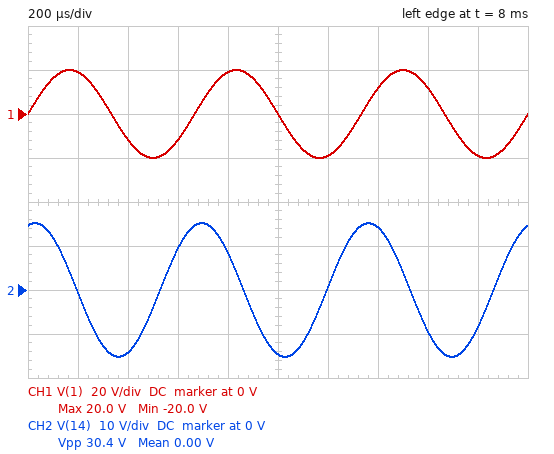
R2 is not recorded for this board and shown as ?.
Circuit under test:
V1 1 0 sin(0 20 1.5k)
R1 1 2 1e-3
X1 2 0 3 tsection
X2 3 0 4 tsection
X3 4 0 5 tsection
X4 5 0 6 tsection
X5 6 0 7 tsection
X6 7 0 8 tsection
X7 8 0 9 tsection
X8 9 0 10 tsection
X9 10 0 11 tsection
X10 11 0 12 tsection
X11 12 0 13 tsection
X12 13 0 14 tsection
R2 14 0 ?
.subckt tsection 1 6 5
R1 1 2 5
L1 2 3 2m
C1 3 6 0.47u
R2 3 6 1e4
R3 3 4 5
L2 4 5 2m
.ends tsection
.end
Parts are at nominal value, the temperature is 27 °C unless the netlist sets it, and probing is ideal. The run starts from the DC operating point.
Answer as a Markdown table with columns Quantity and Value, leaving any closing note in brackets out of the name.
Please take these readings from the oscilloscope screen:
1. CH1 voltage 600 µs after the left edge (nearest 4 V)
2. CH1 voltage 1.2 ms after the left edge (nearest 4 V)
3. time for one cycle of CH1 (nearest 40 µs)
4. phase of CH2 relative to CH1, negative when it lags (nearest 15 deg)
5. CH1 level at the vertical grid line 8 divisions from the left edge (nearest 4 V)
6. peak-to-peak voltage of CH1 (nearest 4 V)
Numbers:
| Quantity | Value |
|---|---|
| CH1 voltage 600 µs after the left edge | -12 V |
| CH1 voltage 1.2 ms after the left edge | -20 V |
| time for one cycle of CH1 | 680 µs |
| phase of CH2 relative to CH1, negative when it lags | 75 deg |
| CH1 level at the vertical grid line 8 divisions from the left edge | 12 V |
| peak-to-peak voltage of CH1 | 40 V |
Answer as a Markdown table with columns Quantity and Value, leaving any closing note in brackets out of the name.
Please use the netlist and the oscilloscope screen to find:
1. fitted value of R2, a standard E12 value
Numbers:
| Quantity | Value |
|---|---|
| fitted value of R2, a standard E12 value | 220 Ω |
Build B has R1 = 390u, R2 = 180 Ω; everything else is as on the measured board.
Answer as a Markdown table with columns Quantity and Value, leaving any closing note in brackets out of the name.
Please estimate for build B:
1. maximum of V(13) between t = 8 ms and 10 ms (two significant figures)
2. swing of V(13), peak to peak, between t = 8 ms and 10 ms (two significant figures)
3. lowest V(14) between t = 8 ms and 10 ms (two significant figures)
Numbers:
| Quantity | Value |
|---|---|
| maximum of V(13) between t = 8 ms and 10 ms | 14 V |
| swing of V(13), peak to peak, between t = 8 ms and 10 ms | 28 V |
| lowest V(14) between t = 8 ms and 10 ms | -14 V |
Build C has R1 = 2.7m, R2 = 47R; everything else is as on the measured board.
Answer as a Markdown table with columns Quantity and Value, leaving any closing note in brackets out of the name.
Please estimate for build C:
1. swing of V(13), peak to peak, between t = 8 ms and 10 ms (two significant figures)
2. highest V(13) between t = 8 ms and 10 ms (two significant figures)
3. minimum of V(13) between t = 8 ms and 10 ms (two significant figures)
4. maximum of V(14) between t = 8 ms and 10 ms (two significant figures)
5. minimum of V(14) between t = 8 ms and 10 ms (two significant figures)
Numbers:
| Quantity | Value |
|---|---|
| swing of V(13), peak to peak, between t = 8 ms and 10 ms | 17 V |
| highest V(13) between t = 8 ms and 10 ms | 8.5 V |
| minimum of V(13) between t = 8 ms and 10 ms | -8.5 V |
| maximum of V(14) between t = 8 ms and 10 ms | 6.2 V |
| minimum of V(14) between t = 8 ms and 10 ms | -6.2 V |
